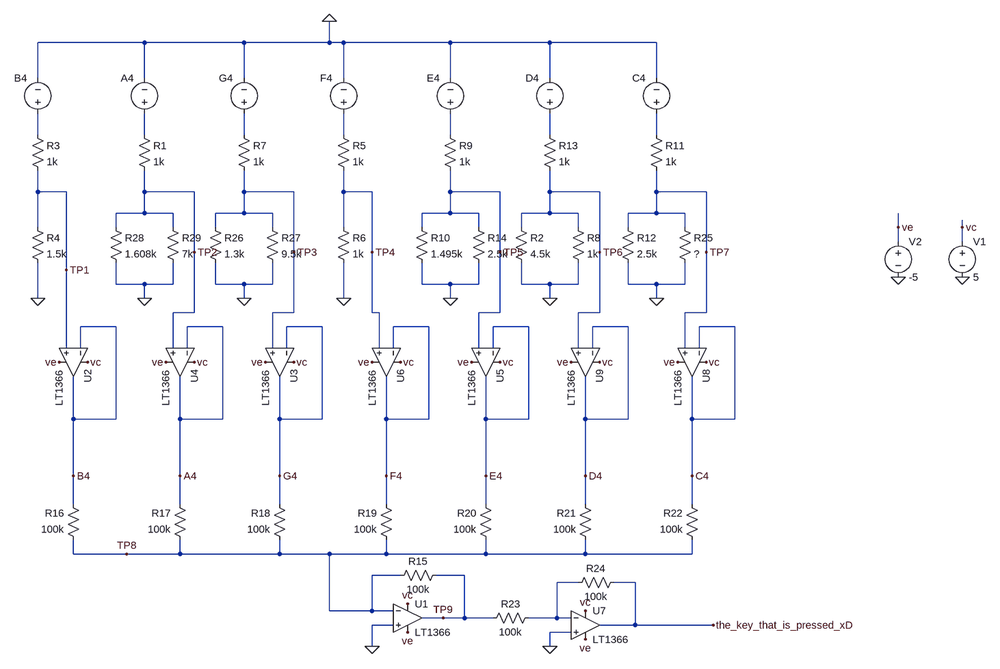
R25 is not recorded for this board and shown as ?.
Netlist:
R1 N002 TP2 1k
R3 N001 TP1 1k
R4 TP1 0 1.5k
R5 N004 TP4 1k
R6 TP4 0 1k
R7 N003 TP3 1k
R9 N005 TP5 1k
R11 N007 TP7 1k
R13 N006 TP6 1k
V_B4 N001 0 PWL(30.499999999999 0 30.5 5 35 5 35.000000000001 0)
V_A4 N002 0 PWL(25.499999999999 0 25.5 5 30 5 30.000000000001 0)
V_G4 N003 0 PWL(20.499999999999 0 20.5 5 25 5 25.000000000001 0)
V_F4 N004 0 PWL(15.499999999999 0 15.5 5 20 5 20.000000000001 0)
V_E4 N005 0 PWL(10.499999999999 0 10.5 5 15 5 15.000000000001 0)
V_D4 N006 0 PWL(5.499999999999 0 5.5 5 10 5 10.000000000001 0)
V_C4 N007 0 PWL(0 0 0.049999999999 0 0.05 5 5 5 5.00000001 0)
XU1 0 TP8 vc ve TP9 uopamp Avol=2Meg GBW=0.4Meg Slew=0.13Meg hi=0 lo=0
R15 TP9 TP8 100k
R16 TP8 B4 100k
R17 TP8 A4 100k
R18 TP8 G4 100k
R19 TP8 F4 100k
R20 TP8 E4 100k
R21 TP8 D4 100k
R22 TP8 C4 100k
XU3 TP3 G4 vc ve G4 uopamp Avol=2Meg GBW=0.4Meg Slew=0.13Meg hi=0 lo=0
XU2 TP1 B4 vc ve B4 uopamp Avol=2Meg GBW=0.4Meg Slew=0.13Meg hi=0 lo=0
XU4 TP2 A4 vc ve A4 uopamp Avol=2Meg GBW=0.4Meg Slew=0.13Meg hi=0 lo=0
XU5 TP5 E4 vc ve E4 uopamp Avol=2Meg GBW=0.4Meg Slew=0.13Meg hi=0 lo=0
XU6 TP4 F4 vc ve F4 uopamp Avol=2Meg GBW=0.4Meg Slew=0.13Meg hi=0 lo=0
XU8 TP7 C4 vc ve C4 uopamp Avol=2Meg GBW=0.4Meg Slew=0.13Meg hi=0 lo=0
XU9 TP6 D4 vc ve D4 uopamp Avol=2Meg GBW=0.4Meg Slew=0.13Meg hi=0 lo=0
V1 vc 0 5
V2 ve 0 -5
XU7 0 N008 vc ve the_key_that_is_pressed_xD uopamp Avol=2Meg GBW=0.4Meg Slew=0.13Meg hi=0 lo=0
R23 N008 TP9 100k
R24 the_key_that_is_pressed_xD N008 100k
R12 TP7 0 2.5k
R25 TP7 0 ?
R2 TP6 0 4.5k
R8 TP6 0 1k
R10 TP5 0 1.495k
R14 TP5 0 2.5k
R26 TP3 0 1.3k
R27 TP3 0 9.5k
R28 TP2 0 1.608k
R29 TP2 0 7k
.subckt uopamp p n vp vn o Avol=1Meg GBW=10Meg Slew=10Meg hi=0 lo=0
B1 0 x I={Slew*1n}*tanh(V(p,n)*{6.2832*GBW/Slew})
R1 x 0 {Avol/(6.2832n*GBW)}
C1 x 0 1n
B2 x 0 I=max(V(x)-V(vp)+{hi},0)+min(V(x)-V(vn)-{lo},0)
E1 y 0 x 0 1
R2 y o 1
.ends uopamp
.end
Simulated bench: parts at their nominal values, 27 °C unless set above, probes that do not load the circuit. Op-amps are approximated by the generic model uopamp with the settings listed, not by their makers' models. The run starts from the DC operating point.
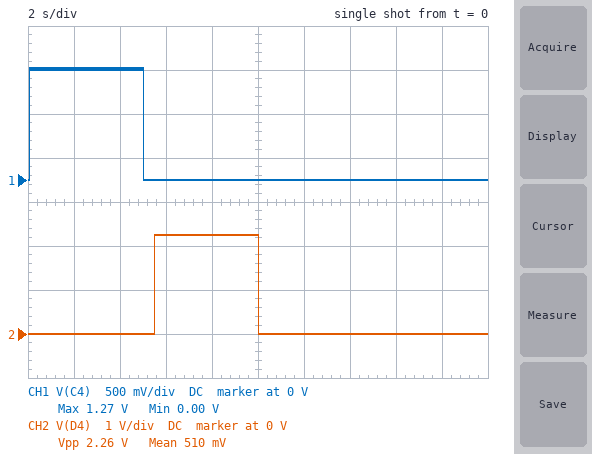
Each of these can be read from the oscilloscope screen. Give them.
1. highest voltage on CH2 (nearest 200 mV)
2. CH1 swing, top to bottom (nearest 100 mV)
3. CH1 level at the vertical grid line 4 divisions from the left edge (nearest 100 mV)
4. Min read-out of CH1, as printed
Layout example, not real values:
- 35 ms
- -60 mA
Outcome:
- 2.2 V
- 1.3 V
- 0 V
- 0.00 V
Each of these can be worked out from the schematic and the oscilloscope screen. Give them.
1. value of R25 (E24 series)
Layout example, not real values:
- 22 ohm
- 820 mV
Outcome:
- 390 Ω
